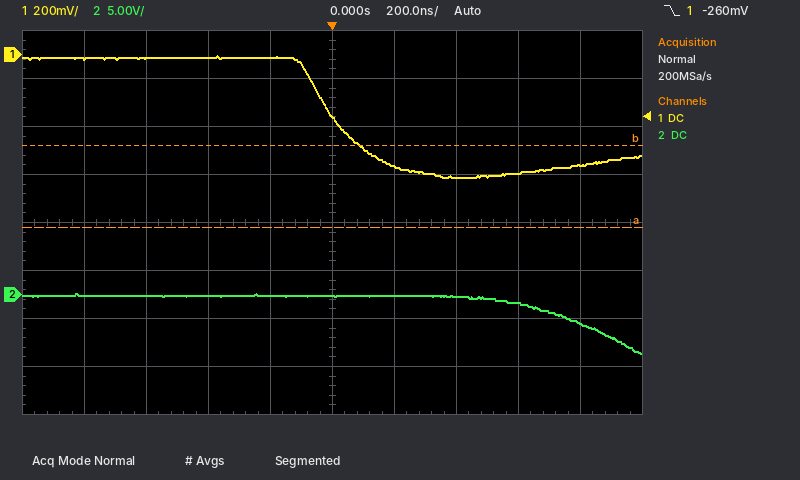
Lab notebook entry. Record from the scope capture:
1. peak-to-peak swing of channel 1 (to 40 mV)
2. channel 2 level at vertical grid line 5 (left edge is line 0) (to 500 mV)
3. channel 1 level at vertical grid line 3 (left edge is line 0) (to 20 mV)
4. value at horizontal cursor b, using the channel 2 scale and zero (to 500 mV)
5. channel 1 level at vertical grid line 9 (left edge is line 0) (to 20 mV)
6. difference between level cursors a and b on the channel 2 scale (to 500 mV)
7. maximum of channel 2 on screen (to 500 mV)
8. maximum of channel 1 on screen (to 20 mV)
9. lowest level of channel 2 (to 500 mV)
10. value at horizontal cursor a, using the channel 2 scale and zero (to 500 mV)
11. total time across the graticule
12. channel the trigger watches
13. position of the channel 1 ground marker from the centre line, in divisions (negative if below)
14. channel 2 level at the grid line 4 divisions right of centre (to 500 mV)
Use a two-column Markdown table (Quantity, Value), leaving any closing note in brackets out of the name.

| Quantity | Value |
|---|---|
| peak-to-peak swing of channel 1 | 520 mV |
| channel 2 level at vertical grid line 5 (left edge is line 0) | 0.0 V |
| channel 1 level at vertical grid line 3 (left edge is line 0) | -20 mV |
| value at horizontal cursor b, using the channel 2 scale and zero | 15.5 V |
| channel 1 level at vertical grid line 9 (left edge is line 0) | -460 mV |
| difference between level cursors a and b on the channel 2 scale | 8.5 V |
| maximum of channel 2 on screen | 0.0 V |
| maximum of channel 1 on screen | 0 mV |
| lowest level of channel 2 | -6.0 V |
| value at horizontal cursor a, using the channel 2 scale and zero | 7.0 V |
| total time across the graticule | 2 µs |
| channel the trigger watches | channel 1 |
| position of the channel 1 ground marker from the centre line, in divisions | +3.5 div |
| channel 2 level at the grid line 4 divisions right of centre | -3.0 V |
